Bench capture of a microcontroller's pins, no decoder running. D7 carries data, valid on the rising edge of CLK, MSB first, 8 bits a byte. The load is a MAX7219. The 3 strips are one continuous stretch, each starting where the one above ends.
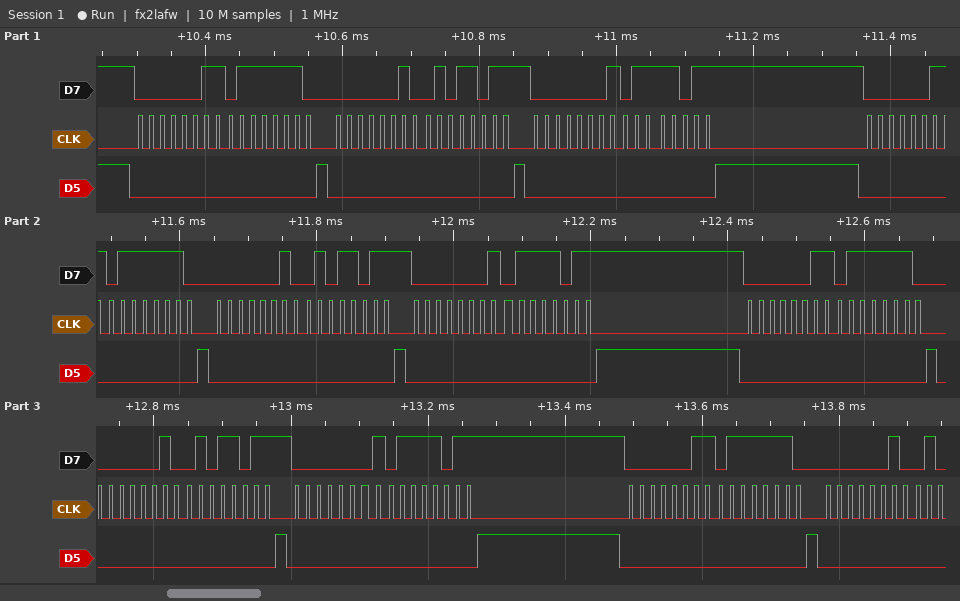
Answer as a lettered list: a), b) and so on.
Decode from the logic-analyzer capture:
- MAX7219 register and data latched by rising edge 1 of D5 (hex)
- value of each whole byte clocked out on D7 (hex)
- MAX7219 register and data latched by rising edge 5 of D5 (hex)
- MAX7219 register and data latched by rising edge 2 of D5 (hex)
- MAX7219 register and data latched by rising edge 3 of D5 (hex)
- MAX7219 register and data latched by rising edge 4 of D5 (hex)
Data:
a) register 0x3, data 0x7E
b) 03 7E 02 5B 01 7B 03 7E 02 5B 01 7B 03 7E 02 5B 01 7B 03 7E 02
c) register 0x2, data 0x5B
d) register 0x2, data 0x5B
e) register 0x1, data 0x7B
f) register 0x3, data 0x7E
